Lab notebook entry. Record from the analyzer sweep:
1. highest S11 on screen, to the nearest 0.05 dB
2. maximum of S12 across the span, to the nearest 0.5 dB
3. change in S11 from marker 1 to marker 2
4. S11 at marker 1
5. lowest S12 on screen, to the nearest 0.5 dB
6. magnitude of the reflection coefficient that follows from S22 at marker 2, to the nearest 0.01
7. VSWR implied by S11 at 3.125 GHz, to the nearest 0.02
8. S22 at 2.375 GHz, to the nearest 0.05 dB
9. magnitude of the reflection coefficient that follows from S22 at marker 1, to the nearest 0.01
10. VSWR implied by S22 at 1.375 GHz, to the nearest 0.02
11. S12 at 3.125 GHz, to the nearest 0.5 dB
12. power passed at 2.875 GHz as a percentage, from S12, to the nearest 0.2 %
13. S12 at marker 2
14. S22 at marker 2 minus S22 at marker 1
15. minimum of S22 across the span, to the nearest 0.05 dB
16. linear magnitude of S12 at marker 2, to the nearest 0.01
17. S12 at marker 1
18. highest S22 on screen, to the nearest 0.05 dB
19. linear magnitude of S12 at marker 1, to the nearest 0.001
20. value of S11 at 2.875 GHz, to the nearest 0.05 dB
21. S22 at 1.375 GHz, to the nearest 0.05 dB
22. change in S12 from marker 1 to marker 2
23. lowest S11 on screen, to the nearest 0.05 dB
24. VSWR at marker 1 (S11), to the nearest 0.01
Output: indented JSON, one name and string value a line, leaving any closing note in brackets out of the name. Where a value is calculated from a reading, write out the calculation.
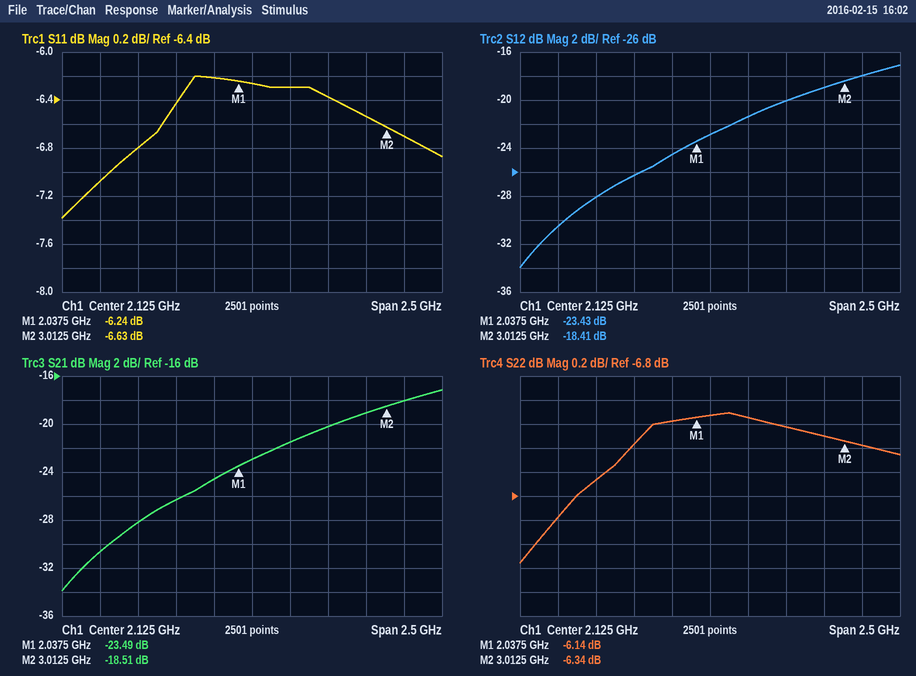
{
  "highest S11 on screen, to the nearest 0.05 dB": "-6.20 dB",
  "maximum of S12 across the span, to the nearest 0.5 dB": "-17.0 dB",
  "change in S11 from marker 1 to marker 2": "-6.63 − (-6.24) = -0.39 dB",
  "S11 at marker 1": "-6.24 dB",
  "lowest S12 on screen, to the nearest 0.5 dB": "-34.0 dB",
  "magnitude of the reflection coefficient that follows from S22 at marker 2, to the nearest 0.01": "10^(-6.34/20) ≈ 0.48",
  "VSWR implied by S11 at 3.125 GHz, to the nearest 0.02": "|Γ| = 10^(-6.7/20) = 0.4624; VSWR = (1 + 0.4624)/(1 − 0.4624) ≈ 2.72",
  "S22 at 2.375 GHz, to the nearest 0.05 dB": "-6.15 dB",
  "magnitude of the reflection coefficient that follows from S22 at marker 1, to the nearest 0.01": "10^(-6.14/20) ≈ 0.49",
  "VSWR implied by S22 at 1.375 GHz, to the nearest 0.02": "|Γ| = 10^(-6.65/20) = 0.4651; VSWR = (1 + 0.4651)/(1 − 0.4651) ≈ 2.74",
  "S12 at 3.125 GHz, to the nearest 0.5 dB": "-18.0 dB",
  "power passed at 2.875 GHz as a percentage, from S12, to the nearest 0.2 %": "10^(-19/10) ≈ 1.26 %, so 1.2 % to the nearest 0.2 %",
  "S12 at marker 2": "-18.41 dB",
  "S22 at marker 2 minus S22 at marker 1": "-6.34 − (-6.14) = -0.20 dB",
  "minimum of S22 across the span, to the nearest 0.05 dB": "-7.35 dB",
  "linear magnitude of S12 at marker 2, to the nearest 0.01": "10^(-18.41/20) ≈ 0.12",
  "S12 at marker 1": "-23.43 dB",
  "highest S22 on screen, to the nearest 0.05 dB": "-6.10 dB",
  "linear magnitude of S12 at marker 1, to the nearest 0.001": "10^(-23.43/20) ≈ 0.067",
  "value of S11 at 2.875 GHz, to the nearest 0.05 dB": "-6.55 dB",
  "S22 at 1.375 GHz, to the nearest 0.05 dB": "-6.65 dB",
  "change in S12 from marker 1 to marker 2": "-18.41 − (-23.43) = 5.02 dB",
  "lowest S11 on screen, to the nearest 0.05 dB": "-7.40 dB",
  "VSWR at marker 1 (S11), to the nearest 0.01": "(1 + 0.4875)/(1 − 0.4875) ≈ 2.90"
}
